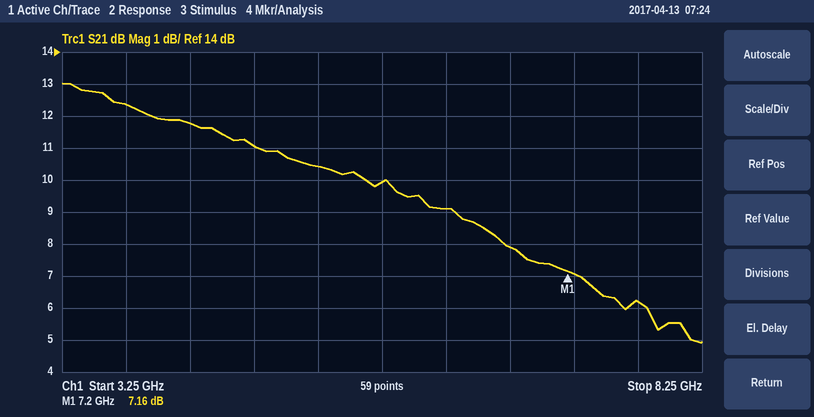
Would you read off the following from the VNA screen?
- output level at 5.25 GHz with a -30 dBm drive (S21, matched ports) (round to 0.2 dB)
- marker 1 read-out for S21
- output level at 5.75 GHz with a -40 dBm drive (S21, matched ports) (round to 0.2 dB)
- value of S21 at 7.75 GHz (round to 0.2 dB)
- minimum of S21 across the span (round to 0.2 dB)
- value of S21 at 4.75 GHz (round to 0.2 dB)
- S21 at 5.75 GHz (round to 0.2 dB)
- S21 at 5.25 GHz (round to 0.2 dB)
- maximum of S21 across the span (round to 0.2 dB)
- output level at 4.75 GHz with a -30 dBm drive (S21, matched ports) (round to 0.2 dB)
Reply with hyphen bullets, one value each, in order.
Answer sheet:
- -19.6 dBm
- 7.16 dB
- -30.0 dBm
- 6.2 dB
- 5.0 dB
- 11.0 dB
- 10.0 dB
- 10.4 dB
- 13.0 dB
- -19.0 dBm
